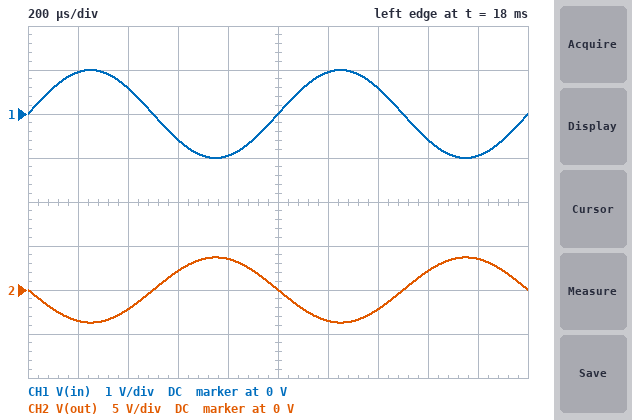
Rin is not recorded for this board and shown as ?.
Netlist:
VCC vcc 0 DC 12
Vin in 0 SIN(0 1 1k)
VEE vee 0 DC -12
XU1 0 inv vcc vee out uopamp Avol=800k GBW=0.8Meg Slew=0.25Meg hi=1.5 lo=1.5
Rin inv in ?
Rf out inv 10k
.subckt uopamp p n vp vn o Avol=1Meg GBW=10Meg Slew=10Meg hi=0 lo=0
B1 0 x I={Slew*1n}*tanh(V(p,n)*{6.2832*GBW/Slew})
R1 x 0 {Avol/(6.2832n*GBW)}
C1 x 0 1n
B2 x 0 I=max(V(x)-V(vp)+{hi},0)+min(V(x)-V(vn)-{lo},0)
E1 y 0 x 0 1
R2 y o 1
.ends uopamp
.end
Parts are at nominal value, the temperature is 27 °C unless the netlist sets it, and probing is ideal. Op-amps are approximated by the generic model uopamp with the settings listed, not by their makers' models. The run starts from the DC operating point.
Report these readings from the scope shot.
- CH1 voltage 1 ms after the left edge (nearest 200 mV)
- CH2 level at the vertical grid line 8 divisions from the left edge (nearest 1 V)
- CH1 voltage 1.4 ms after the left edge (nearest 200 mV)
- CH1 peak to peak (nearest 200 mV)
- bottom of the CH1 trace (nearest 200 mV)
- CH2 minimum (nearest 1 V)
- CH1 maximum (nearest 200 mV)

0 V
2 V
600 mV
2.0 V
-1.0 V
-4 V
1.0 V
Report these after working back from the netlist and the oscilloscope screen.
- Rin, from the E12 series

2.7 kΩ
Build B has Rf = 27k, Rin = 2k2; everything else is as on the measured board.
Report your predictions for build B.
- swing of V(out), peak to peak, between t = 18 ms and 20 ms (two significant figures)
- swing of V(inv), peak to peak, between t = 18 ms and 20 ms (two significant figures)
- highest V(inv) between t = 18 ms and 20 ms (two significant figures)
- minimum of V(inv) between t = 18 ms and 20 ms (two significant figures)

21 V
270 mV
130 mV
-130 mV
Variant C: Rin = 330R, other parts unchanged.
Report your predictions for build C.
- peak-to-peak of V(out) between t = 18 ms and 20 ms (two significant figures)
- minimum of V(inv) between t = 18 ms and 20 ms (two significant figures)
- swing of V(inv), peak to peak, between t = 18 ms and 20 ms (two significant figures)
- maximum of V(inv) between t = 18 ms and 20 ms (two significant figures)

21 V
-630 mV
1.3 V
630 mV
